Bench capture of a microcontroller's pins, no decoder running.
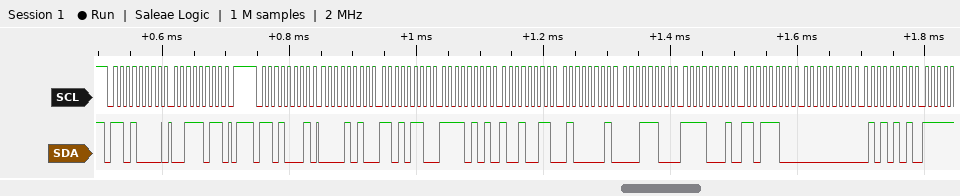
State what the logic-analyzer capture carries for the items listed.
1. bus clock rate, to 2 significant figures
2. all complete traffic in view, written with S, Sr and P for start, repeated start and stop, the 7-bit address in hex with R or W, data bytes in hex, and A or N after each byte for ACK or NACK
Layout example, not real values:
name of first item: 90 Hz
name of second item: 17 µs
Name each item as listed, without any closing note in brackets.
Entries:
bus clock rate, to 2 significant figures: 100 kHz
all complete traffic in view, written with S, Sr and P for start, repeated start and stop, the 7-bit address in hex with R or W, data bytes in hex, and A or N after each byte for ACK or NACK: S 68W A 3B A P S 68R A 0A A D6 A F5 A 93 A 41 A 1C A F1 A DC A 00 A 55 A
